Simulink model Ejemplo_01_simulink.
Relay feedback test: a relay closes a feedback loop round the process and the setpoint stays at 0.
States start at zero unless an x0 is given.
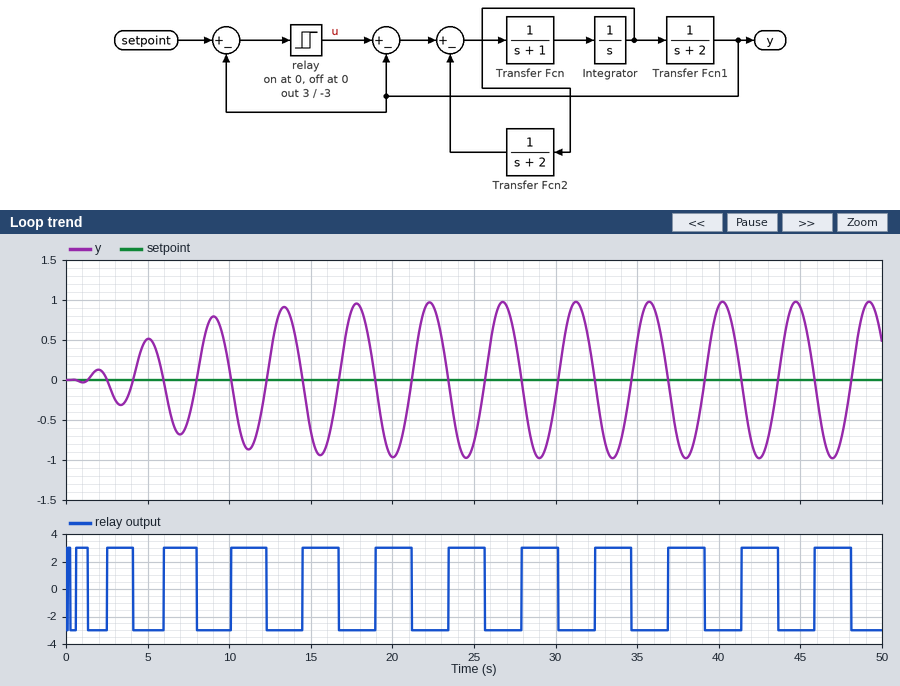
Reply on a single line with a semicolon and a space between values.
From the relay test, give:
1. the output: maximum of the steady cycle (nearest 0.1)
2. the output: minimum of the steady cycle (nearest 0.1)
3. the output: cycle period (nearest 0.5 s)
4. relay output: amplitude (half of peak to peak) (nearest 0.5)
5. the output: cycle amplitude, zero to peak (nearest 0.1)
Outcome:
1.0; -1.0; 4.5 s; 3.0; 1.0
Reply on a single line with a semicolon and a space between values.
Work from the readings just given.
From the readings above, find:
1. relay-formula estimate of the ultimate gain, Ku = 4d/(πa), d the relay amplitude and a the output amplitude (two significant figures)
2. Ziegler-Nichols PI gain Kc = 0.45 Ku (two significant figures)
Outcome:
3.8; 1.7
